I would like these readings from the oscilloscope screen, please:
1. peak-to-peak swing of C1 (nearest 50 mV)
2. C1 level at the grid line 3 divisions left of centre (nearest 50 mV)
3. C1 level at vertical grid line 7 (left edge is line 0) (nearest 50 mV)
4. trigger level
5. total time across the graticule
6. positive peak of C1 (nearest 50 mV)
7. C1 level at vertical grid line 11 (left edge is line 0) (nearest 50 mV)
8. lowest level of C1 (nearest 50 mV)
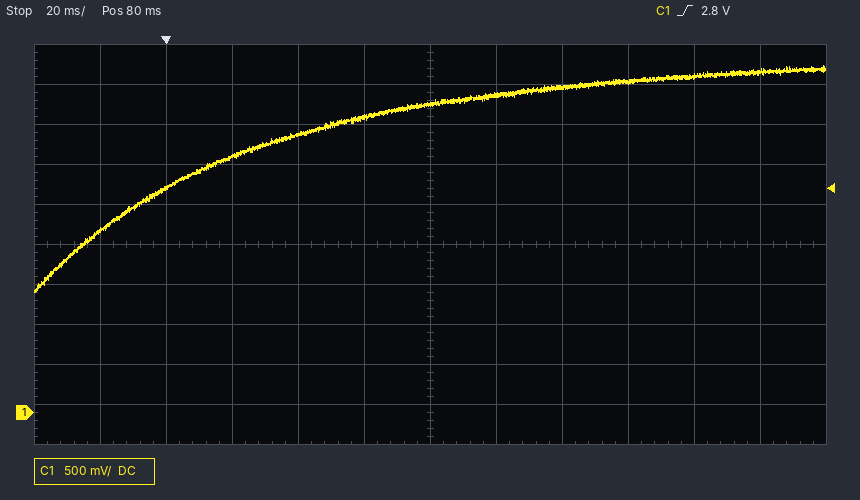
2.85 V
3.20 V
3.95 V
2.8 V
240 ms
4.35 V
4.25 V
1.50 V
